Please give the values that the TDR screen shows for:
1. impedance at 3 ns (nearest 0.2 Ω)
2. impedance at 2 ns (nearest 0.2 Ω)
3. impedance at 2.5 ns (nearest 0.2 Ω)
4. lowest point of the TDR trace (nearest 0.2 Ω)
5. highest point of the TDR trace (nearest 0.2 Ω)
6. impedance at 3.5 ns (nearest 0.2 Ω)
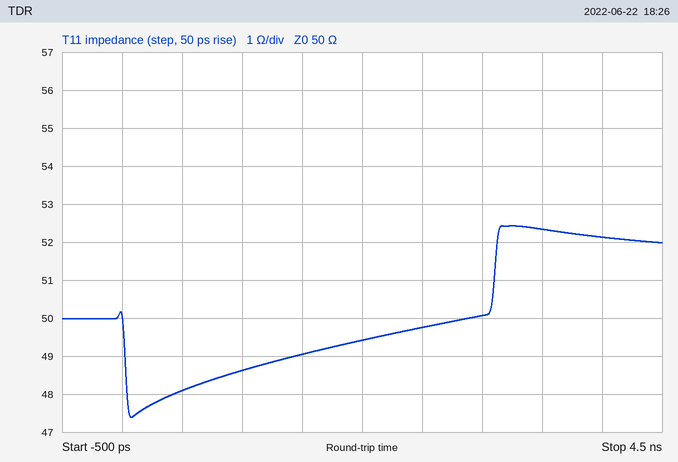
50.0 Ω
49.4 Ω
49.8 Ω
47.4 Ω
52.4 Ω
52.4 Ω
